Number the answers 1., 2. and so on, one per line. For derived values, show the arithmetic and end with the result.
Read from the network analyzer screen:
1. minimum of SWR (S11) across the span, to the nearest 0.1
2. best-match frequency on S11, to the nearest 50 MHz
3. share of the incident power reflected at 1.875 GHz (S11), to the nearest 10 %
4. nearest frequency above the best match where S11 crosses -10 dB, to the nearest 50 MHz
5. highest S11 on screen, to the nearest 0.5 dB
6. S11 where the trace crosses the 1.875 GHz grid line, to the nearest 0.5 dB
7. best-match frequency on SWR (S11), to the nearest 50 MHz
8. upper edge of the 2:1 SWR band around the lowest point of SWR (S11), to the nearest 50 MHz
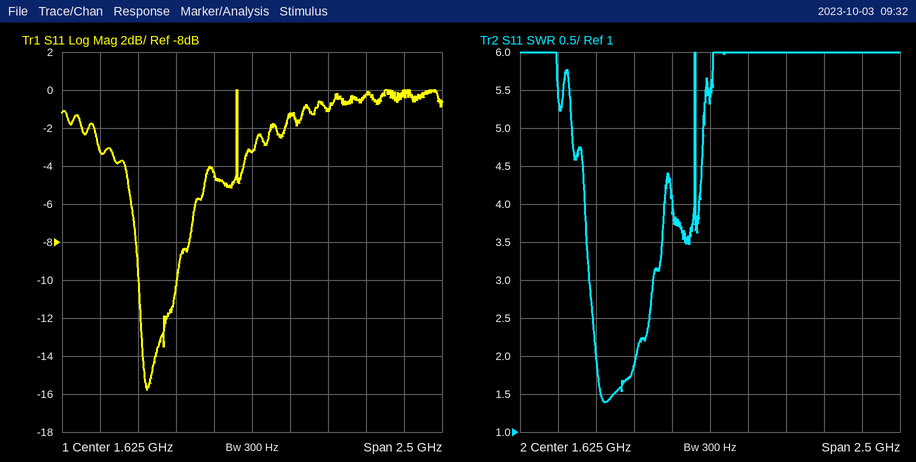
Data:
1. 1.4
2. 950 MHz
3. 10^(-1.5/10) ≈ 70.8 %, so 70 % to the nearest 10 %
4. 1.15 GHz
5. 0.0 dB
6. -1.5 dB
7. 950 MHz
8. 1.15 GHz
